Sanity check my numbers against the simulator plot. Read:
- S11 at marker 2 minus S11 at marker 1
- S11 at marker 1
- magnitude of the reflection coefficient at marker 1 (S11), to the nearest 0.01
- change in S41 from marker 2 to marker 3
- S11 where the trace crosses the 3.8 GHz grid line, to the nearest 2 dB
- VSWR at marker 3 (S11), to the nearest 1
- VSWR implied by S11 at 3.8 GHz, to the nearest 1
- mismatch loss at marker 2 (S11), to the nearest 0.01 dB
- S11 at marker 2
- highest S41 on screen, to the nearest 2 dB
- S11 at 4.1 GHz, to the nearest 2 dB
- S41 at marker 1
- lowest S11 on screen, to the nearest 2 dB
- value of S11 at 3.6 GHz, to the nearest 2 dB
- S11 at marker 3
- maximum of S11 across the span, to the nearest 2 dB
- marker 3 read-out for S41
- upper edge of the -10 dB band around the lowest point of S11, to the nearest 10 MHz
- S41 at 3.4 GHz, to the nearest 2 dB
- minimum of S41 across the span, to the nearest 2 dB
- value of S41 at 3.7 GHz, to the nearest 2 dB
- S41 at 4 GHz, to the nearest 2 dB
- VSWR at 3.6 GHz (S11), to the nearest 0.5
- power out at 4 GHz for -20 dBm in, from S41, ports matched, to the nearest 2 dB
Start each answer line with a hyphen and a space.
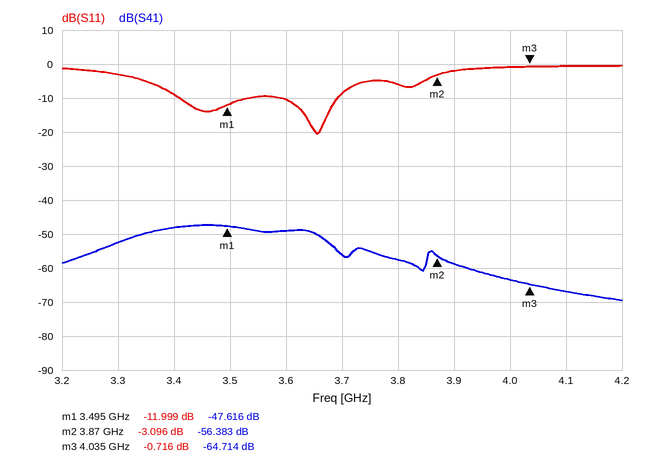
- 8.903 dB
- -11.999 dB
- 0.25
- -8.331 dB
- -6 dB
- 24
- 3
- 2.93 dB
- -3.096 dB
- -48 dB
- 0 dB
- -47.616 dB
- -20 dB
- -10 dB
- -0.716 dB
- 0 dB
- -64.714 dB
- 3.69 GHz
- -48 dB
- -70 dB
- -56 dB
- -64 dB
- 2.0
- -84 dBm
